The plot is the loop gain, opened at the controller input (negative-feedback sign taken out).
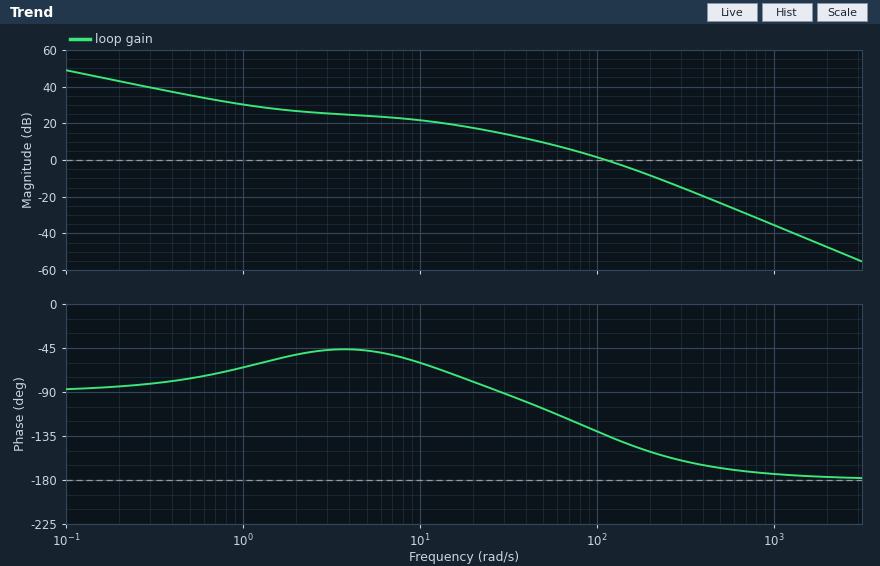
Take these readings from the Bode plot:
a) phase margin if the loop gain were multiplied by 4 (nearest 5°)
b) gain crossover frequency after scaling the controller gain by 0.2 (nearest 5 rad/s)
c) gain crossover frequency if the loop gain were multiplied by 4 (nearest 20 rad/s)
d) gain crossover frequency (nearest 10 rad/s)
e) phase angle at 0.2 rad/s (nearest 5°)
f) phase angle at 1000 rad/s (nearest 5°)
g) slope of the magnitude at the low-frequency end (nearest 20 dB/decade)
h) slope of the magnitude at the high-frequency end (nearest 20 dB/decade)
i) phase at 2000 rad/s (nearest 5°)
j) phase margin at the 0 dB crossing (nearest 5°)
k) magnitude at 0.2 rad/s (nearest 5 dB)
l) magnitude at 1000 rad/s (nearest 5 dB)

25°
30 rad/s
260 rad/s
110 rad/s
-85°
-175°
-20 dB/decade
-40 dB/decade
-175°
45°
45 dB
-35 dB
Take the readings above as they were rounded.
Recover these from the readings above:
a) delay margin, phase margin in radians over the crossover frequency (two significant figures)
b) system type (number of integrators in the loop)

0.0071 s
1
